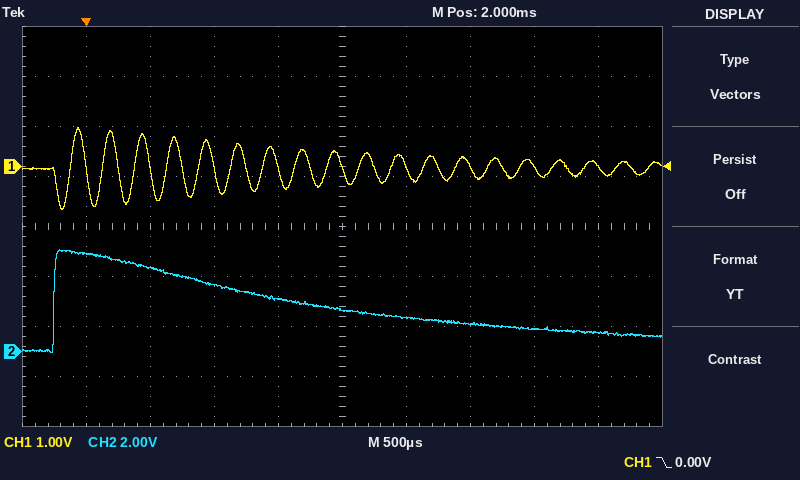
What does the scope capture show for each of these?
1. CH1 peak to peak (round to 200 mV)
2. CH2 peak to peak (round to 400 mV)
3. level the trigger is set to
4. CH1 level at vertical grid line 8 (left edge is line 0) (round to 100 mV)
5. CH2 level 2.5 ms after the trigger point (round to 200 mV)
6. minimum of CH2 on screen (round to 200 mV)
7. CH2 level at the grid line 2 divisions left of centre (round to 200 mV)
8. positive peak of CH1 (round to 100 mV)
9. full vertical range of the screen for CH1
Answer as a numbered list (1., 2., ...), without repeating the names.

1. 1.6 V
2. 4.0 V
3. 0.00 V
4. 0.0 V
5. 1.4 V
6. 0.0 V
7. 2.6 V
8. 800 mV
9. 8 V
